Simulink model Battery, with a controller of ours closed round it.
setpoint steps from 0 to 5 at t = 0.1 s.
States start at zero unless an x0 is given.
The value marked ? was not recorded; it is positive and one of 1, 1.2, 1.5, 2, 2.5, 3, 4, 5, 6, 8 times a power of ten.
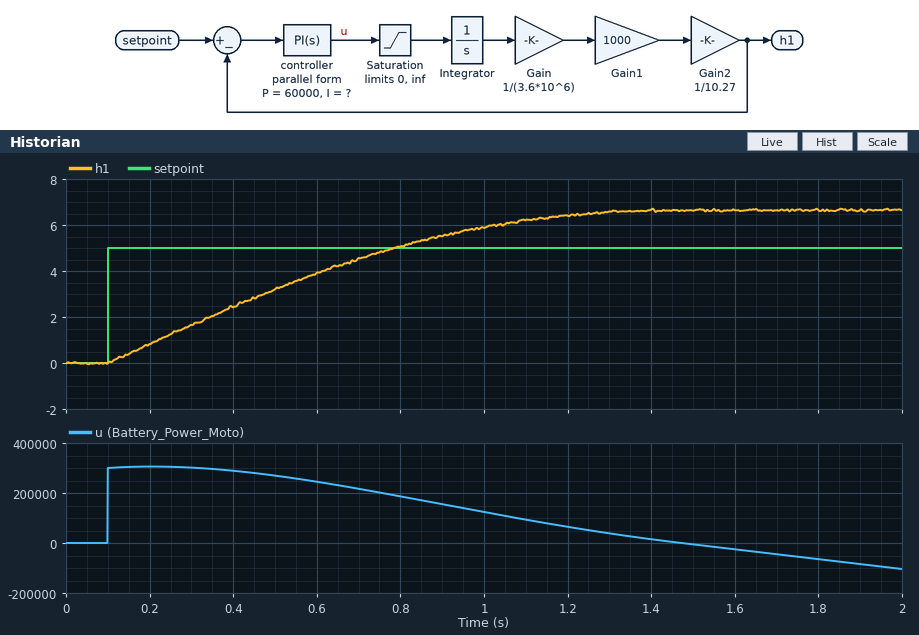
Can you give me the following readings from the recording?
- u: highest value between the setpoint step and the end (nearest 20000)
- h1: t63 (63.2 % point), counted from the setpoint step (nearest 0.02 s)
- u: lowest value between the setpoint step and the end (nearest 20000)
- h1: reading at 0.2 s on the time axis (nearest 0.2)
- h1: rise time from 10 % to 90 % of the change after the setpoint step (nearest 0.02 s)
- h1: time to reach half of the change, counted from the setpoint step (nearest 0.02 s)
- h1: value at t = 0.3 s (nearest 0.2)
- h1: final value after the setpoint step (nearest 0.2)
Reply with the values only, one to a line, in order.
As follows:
300000
0.54 s
-100000
0.8
0.84 s
0.42 s
1.6
6.6
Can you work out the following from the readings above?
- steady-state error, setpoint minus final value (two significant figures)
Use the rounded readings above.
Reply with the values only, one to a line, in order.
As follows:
-1.6
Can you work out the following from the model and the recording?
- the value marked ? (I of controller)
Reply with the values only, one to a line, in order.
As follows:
120000
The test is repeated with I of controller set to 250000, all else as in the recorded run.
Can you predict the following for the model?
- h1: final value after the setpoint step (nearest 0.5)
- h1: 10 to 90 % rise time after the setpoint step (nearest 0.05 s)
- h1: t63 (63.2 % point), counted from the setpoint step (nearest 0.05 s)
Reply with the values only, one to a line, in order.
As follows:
7.0
0.65 s
0.45 s
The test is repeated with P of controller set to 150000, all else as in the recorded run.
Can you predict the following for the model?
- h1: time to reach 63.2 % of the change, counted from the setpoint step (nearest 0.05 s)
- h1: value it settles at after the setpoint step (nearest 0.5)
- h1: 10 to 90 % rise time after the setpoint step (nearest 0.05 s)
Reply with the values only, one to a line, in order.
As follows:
0.25 s
5.5
0.50 s
